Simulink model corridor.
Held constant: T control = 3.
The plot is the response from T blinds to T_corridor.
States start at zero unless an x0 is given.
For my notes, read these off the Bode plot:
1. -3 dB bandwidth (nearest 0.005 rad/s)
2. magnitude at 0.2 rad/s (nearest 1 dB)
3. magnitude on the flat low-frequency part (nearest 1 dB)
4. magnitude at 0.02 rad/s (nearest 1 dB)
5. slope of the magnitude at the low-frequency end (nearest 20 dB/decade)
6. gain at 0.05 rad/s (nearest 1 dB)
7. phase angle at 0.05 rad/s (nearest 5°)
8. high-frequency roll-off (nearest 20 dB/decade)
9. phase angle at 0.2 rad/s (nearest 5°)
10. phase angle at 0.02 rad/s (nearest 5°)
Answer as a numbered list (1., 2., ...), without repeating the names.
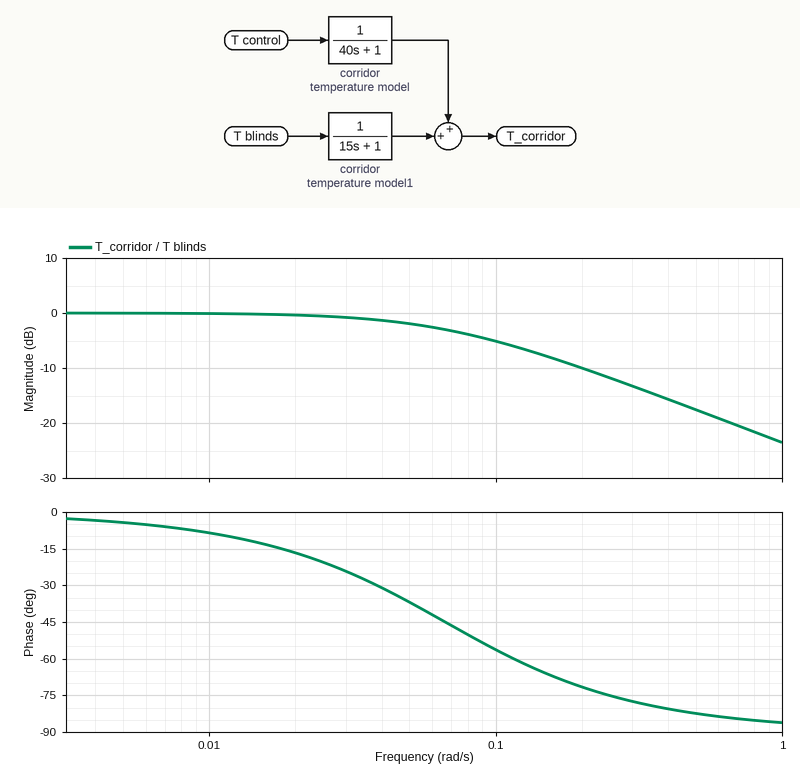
1. 0.065 rad/s
2. -10 dB
3. 0 dB
4. 0 dB
5. 0 dB/decade
6. -2 dB
7. -35°
8. -20 dB/decade
9. -70°
10. -15°
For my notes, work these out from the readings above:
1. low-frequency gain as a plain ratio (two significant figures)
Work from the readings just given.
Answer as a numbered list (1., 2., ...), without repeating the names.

1. 1.0
